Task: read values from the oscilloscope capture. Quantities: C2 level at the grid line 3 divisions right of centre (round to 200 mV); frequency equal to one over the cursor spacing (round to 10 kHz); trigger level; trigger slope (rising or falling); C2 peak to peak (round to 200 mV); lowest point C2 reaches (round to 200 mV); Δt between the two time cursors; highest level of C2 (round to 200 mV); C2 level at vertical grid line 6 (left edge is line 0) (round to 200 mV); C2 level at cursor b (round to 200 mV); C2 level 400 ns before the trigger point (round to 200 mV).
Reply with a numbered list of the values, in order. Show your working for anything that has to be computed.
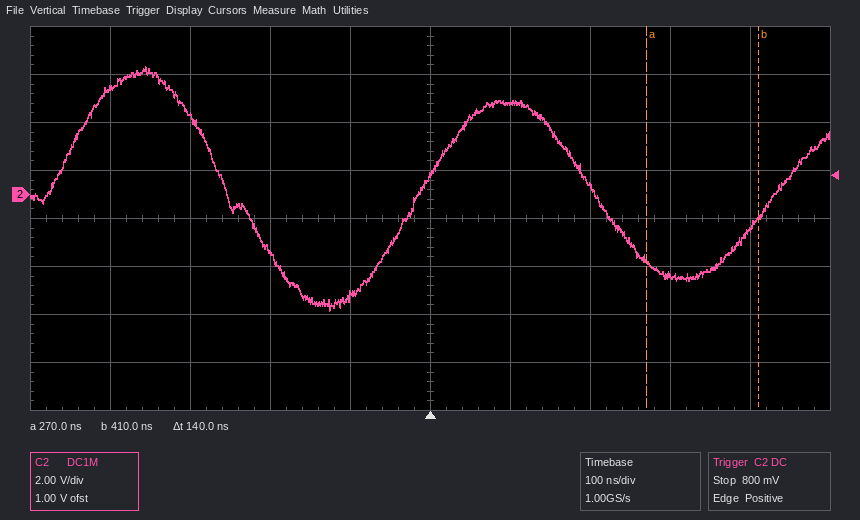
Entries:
1. -3.4 V
2. 1 / 140 ns ≈ 7.14 MHz
3. 800 mV
4. rising
5. 5.4 V − (-4.8 V) = 10.2 V
6. -4.8 V
7. 140 ns
8. 5.4 V
9. 3.8 V
10. -1.0 V
11. 4.4 V
